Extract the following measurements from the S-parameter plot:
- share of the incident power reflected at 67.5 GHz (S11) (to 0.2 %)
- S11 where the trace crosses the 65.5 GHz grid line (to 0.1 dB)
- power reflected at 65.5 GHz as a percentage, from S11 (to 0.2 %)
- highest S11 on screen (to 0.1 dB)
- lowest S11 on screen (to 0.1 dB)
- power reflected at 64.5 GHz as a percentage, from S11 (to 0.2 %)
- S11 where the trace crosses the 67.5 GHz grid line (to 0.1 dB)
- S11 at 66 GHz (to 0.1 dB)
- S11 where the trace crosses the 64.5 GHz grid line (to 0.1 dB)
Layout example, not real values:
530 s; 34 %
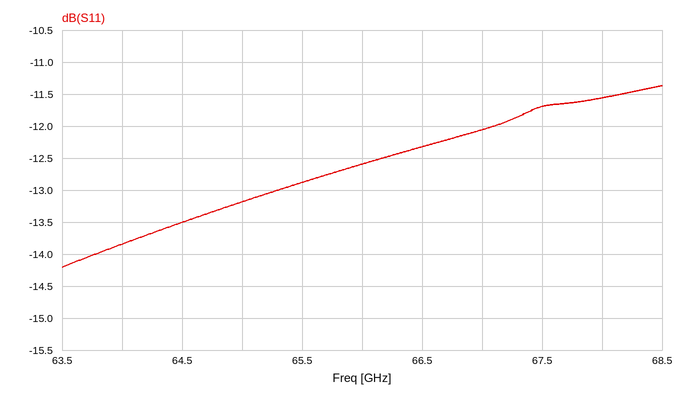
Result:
6.8 %; -12.9 dB; 5.2 %; -11.4 dB; -14.2 dB; 4.4 %; -11.7 dB; -12.6 dB; -13.5 dB
